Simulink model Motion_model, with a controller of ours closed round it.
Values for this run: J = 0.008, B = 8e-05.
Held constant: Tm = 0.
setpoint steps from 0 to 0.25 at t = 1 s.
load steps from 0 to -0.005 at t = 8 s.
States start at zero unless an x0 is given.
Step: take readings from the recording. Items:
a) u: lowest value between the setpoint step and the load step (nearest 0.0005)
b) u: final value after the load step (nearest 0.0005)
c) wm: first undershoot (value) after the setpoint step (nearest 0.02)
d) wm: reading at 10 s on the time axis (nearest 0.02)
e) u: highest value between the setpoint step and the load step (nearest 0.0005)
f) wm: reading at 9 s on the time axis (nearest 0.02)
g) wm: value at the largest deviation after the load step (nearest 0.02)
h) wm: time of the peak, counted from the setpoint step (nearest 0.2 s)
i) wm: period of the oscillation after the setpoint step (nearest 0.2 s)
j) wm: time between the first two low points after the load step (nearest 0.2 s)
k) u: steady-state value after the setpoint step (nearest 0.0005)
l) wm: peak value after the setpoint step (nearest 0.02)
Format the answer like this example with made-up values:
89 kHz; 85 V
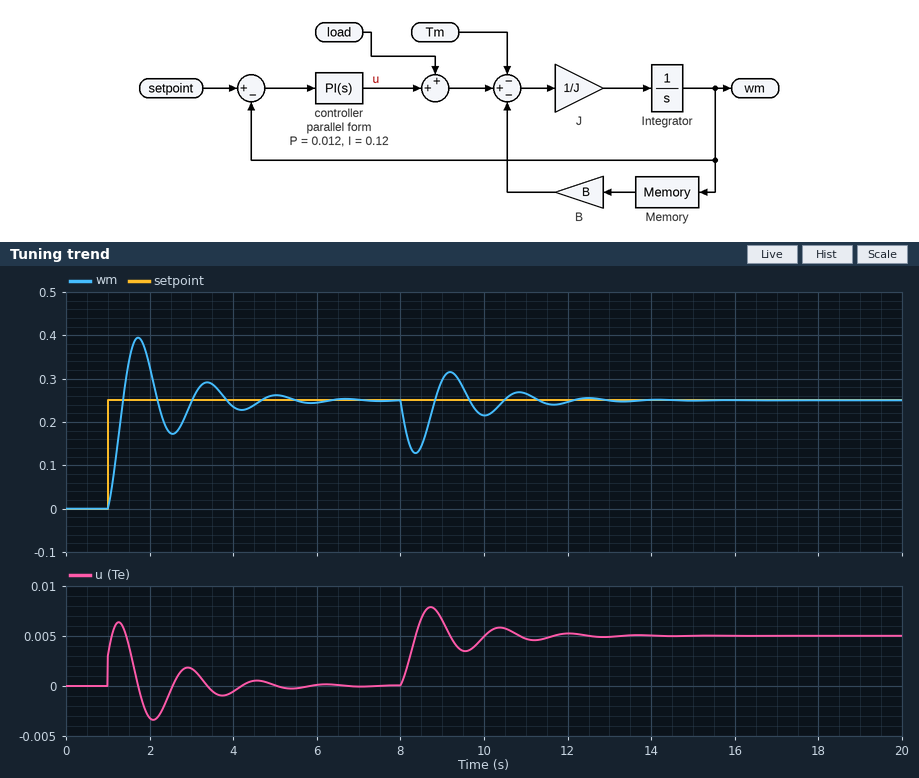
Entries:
-0.0035; 0.0050; 0.18; 0.22; 0.0065; 0.30; 0.12; 0.8 s; 1.6 s; 1.6 s; 0.0000; 0.40
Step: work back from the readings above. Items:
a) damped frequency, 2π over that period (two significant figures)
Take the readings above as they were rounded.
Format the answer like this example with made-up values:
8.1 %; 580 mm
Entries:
3.9 rad/s
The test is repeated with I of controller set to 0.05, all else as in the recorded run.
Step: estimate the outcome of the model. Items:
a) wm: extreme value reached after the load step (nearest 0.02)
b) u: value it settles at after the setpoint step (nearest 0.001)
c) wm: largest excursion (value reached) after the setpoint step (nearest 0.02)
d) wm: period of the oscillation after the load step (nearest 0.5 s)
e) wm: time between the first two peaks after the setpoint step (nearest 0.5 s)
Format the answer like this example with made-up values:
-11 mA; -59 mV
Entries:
0.08; 0.000; 0.36; 2.5 s; 2.5 s
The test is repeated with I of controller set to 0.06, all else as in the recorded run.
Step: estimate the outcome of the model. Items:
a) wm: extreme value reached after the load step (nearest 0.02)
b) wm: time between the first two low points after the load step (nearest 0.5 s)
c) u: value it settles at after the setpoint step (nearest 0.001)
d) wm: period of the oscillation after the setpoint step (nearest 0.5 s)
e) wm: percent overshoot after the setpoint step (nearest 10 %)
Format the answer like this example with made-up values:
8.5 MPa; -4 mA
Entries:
0.10; 2.5 s; 0.000; 2.5 s; 50 %
